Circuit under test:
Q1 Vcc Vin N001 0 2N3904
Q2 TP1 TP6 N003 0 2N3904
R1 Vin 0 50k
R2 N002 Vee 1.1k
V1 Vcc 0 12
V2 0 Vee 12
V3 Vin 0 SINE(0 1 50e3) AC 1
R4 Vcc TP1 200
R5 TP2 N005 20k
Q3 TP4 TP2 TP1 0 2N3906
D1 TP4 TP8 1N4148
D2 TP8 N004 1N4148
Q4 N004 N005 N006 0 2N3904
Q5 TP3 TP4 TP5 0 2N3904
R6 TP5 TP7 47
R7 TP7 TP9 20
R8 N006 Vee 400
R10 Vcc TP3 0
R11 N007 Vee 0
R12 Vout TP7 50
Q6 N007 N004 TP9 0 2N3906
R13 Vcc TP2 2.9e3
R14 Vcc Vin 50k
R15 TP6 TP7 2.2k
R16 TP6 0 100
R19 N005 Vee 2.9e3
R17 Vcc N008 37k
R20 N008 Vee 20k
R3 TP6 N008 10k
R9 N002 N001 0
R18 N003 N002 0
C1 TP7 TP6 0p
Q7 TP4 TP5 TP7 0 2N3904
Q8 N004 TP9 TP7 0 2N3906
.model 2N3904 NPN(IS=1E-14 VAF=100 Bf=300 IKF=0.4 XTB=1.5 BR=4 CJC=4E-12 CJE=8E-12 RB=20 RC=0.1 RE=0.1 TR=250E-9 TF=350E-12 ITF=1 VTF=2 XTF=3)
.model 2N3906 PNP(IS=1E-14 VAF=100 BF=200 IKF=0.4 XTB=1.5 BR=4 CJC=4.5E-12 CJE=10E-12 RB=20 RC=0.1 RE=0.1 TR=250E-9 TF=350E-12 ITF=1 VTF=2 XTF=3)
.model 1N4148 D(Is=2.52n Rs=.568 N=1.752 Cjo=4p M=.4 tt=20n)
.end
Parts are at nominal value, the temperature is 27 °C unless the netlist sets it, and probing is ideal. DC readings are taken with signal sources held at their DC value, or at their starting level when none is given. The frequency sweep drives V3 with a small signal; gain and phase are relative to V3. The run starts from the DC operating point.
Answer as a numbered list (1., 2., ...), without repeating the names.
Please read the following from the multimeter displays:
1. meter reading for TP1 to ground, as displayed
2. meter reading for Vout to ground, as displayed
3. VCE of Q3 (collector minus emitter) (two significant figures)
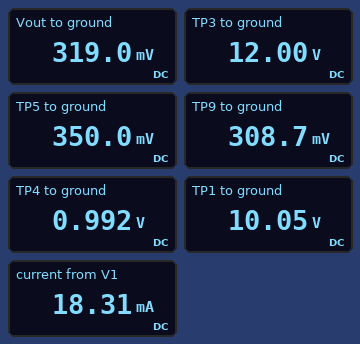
1. 10.05 V
2. 319.0 mV
3. -9.1 V
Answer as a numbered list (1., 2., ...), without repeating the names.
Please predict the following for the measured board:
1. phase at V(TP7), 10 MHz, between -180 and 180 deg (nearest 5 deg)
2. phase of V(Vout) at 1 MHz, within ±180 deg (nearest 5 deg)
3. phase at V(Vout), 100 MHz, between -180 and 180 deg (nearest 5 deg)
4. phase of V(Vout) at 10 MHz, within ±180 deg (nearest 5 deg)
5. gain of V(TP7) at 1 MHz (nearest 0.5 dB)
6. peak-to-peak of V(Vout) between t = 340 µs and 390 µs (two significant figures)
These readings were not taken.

1. -45 deg
2. -5 deg
3. -115 deg
4. -45 deg
5. 27.0 dB
6. 20 V
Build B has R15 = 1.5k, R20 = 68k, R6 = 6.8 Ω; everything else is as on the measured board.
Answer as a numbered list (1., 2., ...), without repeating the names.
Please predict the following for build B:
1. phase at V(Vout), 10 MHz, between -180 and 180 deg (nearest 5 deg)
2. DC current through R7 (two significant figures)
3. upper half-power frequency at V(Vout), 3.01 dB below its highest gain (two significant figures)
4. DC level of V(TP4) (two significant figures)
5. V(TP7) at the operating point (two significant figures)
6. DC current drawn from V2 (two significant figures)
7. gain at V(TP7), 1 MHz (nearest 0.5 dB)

1. -35 deg
2. 890 µA
3. 21 MHz
4. 480 mV
5. -170 mV
6. 18 mA
7. 24.0 dB
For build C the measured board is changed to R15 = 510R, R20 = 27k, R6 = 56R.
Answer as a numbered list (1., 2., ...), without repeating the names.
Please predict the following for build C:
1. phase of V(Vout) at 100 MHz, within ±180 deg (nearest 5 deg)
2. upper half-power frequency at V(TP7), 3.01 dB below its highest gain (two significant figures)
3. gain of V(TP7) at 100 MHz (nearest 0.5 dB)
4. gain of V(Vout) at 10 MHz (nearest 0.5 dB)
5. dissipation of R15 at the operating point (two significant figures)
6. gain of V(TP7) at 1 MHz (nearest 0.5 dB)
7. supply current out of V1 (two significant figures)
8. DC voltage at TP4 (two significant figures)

1. -100 deg
2. 42 MHz
3. 2.5 dB
4. 16.0 dB
5. 2.1 µW
6. 15.5 dB
7. 18 mA
8. 700 mV
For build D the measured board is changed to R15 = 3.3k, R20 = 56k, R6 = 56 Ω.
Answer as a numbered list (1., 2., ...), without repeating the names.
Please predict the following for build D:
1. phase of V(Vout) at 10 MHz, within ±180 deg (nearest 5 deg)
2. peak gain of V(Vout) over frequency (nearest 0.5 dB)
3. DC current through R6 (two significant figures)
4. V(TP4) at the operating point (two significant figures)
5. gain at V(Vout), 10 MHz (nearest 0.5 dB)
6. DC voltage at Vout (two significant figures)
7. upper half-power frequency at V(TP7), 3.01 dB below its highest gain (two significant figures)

1. -60 deg
2. 30.5 dB
3. 530 µA
4. 380 mV
5. 27.5 dB
6. -280 mV
7. 10 MHz
